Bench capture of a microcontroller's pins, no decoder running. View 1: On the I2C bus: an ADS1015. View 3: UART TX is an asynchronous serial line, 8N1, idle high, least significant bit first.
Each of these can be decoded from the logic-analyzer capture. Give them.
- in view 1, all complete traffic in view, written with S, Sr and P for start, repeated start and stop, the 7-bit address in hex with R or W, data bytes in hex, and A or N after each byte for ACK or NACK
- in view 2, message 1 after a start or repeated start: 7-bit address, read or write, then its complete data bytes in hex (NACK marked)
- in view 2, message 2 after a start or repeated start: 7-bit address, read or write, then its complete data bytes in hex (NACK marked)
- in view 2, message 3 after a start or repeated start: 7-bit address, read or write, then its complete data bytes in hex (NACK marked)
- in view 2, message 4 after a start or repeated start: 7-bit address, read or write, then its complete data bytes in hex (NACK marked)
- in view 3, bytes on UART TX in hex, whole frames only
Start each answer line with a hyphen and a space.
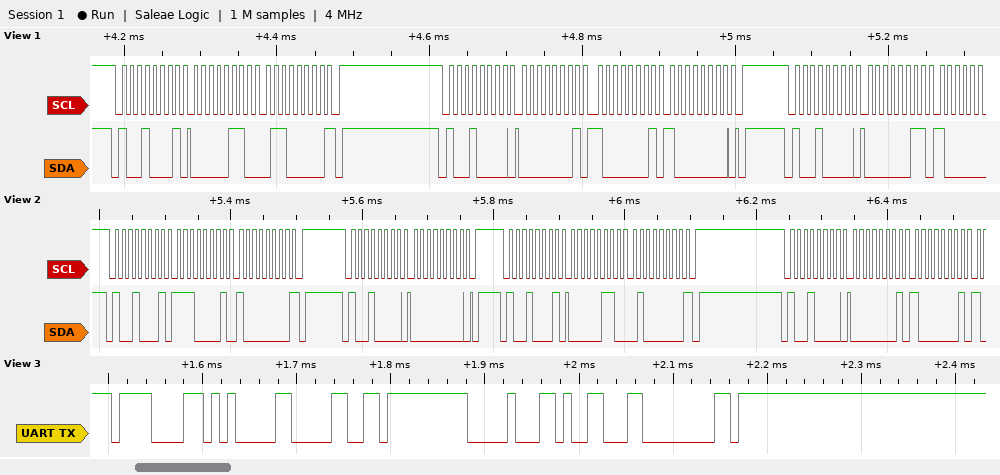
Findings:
- S 48R A 06 A 60 N P S 48W A 01 A 81 A 80 A P S 48W A 03 A
- 0x48 read: E1 80 NACK
- 0x48 write: 00
- 0x48 read: 06 40 NACK
- 0x48 write: 01 81
- 0F 05 30 FF 10 19 00 FF
